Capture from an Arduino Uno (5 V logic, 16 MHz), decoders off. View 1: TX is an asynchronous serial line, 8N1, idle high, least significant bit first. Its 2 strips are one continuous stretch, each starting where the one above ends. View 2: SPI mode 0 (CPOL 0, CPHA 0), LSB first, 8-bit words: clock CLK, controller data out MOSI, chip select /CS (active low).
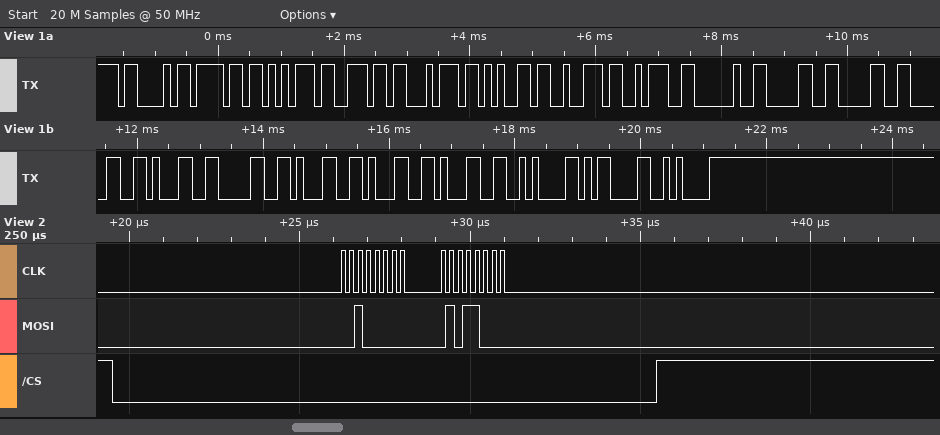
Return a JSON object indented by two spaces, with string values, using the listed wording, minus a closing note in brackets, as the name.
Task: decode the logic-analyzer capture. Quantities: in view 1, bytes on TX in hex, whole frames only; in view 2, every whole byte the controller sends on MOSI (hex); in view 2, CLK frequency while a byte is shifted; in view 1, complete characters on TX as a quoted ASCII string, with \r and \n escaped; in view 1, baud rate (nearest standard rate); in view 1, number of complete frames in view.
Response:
{
  "in view 1, bytes on TX in hex, whole frames only": "43 6F 75 6E 74 65 72 3A 20 30 30 30 31 30 31 31 31 0A 0D 0A",
  "in view 2, every whole byte the controller sends on MOSI": "04 1A",
  "in view 2, CLK frequency while a byte is shifted": "4 MHz",
  "in view 1, complete characters on TX as a quoted ASCII string, with \\r and \\n escaped": "\"Counter: 00010111\\n\\r\\n\"",
  "in view 1, baud rate": "9600 baud",
  "in view 1, number of complete frames in view": "20"
}
